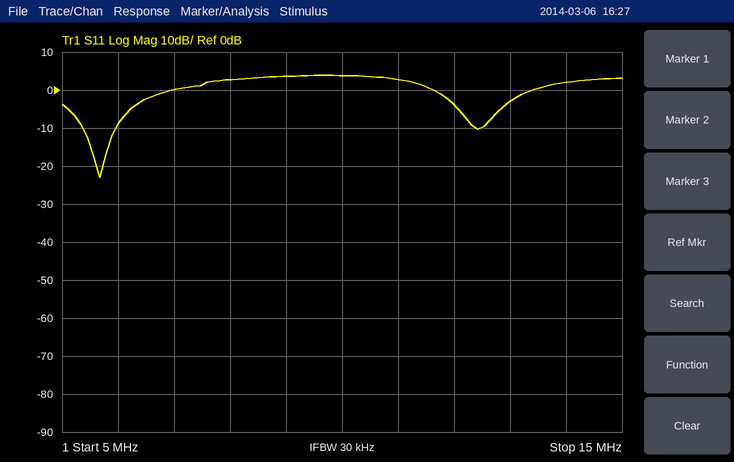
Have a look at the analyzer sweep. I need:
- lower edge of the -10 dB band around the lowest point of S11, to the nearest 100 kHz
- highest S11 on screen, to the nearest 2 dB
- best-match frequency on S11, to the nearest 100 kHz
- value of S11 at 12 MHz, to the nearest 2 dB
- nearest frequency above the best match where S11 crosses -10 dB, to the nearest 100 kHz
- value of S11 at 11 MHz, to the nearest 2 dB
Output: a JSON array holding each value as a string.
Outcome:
["5.4 MHz", "4 dB", "5.7 MHz", "-4 dB", "6.0 MHz", "2 dB"]
